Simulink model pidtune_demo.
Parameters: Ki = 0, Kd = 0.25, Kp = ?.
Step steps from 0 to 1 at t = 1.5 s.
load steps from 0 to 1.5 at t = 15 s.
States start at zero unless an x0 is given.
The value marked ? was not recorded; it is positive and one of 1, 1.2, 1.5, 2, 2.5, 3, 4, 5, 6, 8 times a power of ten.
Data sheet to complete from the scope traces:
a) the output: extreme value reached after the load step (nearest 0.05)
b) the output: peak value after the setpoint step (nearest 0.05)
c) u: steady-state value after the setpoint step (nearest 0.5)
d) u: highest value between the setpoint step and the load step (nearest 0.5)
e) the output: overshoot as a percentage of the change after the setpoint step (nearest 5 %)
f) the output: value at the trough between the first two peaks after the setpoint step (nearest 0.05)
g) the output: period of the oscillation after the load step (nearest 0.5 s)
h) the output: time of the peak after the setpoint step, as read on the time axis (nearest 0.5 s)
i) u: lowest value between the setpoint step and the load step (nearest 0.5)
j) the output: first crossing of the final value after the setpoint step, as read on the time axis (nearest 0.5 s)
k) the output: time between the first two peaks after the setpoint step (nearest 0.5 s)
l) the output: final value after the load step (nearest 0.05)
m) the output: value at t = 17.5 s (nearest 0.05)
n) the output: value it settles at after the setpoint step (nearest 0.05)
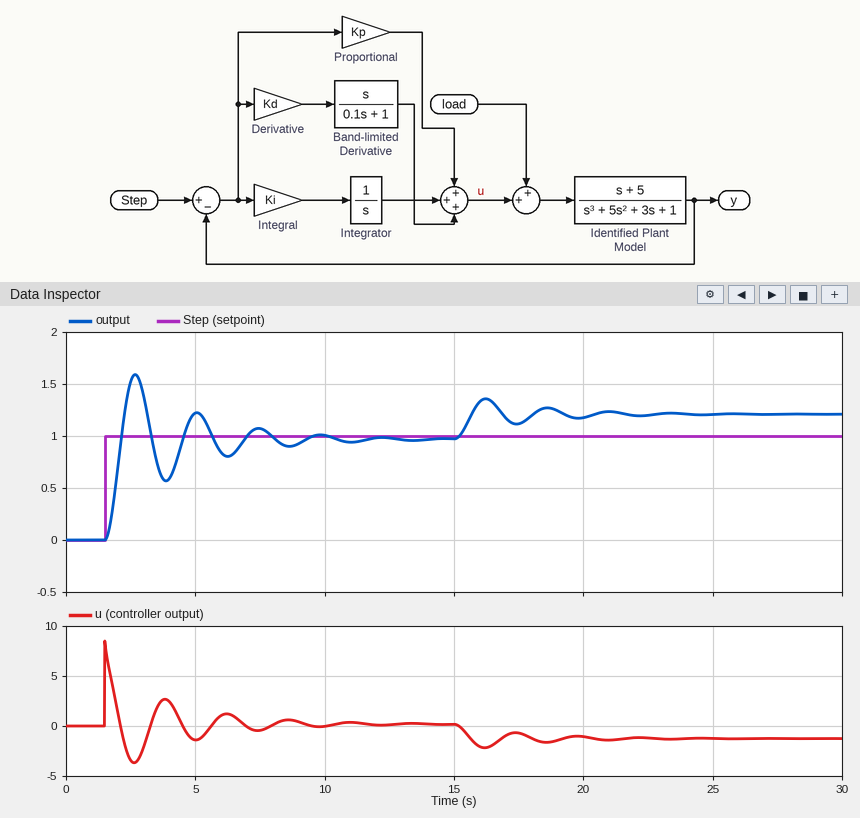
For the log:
1.35
1.60
0.0
8.5
65 %
0.55
2.5 s
2.5 s
-3.5
2.0 s
2.5 s
1.20
1.10
0.95
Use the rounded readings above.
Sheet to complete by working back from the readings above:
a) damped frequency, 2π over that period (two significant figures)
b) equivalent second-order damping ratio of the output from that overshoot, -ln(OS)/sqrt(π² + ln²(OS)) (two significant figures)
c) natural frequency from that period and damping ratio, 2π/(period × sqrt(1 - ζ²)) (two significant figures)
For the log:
2.5 rad/s
0.14
2.5 rad/s
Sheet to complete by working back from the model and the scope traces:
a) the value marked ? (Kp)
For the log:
6
